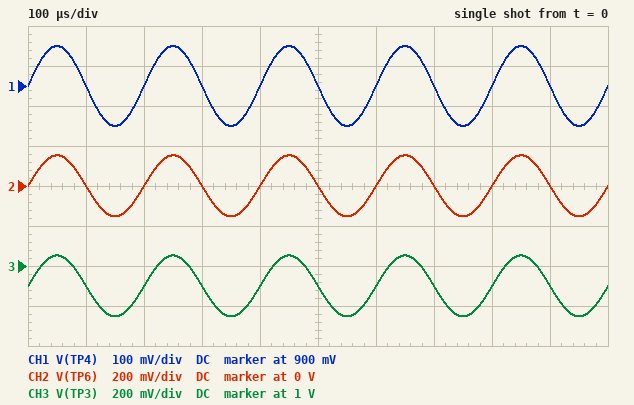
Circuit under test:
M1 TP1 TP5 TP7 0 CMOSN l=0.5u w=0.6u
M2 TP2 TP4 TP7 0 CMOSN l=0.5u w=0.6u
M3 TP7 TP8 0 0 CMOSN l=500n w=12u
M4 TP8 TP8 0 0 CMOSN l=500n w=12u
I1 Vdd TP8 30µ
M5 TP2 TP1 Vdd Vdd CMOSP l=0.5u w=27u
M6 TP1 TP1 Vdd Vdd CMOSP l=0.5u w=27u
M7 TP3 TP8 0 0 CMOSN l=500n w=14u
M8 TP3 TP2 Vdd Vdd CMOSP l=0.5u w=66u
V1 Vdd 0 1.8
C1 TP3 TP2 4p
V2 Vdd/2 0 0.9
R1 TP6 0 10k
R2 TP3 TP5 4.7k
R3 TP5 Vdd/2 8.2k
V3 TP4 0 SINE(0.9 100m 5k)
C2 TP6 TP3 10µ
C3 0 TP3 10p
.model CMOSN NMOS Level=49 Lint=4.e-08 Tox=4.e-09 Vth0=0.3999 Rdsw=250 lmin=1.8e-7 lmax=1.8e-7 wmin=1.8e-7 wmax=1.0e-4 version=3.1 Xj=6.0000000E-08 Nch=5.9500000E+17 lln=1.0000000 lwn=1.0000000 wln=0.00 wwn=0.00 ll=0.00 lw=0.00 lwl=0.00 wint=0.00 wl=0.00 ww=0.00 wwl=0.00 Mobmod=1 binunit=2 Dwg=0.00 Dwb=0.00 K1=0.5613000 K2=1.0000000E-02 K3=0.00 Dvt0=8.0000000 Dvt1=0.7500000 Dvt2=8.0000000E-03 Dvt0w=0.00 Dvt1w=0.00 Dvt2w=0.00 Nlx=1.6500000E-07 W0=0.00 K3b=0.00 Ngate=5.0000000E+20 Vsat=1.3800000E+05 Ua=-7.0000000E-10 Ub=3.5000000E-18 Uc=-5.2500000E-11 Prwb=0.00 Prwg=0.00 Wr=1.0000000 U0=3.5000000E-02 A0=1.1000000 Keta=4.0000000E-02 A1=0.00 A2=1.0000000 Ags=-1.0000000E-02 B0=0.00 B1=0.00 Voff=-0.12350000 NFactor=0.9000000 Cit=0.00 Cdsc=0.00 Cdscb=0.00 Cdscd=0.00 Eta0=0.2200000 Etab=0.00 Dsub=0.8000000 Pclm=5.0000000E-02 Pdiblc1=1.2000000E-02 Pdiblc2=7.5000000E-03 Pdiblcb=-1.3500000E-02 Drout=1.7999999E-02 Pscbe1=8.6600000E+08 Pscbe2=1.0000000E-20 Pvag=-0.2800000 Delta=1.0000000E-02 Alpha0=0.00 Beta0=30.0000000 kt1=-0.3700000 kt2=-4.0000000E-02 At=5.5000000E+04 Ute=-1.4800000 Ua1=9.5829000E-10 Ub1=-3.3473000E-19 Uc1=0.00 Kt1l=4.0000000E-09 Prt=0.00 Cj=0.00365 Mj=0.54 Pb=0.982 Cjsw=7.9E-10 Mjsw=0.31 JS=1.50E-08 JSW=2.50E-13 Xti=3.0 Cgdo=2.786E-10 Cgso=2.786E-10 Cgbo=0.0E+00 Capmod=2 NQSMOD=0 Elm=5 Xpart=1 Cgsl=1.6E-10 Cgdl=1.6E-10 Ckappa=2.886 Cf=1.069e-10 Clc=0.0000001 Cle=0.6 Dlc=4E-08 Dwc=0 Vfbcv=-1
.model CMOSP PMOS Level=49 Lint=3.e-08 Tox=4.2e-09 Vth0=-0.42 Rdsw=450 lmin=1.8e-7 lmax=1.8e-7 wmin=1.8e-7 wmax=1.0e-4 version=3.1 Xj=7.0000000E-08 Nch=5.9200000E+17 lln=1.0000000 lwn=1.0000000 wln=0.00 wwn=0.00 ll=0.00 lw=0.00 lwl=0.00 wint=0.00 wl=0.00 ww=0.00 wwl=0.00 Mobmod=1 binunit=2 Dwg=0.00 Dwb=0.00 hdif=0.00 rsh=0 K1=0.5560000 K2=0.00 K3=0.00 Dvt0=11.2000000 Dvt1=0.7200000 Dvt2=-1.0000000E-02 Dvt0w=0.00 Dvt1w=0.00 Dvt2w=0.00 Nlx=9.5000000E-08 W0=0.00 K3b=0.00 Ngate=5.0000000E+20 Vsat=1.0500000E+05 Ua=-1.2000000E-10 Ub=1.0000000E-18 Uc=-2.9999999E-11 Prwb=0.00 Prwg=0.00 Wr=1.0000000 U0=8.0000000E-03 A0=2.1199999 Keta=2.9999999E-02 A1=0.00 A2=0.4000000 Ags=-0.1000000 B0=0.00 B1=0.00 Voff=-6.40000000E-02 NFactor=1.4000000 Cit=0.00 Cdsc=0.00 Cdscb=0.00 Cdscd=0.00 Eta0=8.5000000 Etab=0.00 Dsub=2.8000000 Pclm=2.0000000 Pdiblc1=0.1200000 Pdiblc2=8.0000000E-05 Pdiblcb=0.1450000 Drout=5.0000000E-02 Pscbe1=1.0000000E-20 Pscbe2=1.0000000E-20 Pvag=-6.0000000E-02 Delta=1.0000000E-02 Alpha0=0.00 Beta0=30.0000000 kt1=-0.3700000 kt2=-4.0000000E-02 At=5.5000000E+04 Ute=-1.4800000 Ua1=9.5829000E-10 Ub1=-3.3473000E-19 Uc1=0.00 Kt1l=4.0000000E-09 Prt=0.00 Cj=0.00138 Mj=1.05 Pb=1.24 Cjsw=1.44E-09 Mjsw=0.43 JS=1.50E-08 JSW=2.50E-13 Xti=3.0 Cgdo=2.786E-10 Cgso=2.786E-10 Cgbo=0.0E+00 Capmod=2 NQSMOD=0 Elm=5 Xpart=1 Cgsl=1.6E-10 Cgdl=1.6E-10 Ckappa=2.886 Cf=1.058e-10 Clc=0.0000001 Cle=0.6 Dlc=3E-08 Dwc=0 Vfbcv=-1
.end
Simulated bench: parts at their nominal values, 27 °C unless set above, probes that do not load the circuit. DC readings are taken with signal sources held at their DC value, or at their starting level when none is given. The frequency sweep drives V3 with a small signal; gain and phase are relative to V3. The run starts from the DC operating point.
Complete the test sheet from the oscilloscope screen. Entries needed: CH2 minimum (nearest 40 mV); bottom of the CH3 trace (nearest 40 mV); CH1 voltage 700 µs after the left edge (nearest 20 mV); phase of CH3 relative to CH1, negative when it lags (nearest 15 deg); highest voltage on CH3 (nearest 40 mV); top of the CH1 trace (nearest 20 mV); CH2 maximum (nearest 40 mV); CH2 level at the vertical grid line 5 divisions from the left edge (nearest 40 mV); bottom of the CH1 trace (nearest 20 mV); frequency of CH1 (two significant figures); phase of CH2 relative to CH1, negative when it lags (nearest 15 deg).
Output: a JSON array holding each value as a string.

["-160 mV", "760 mV", "900 mV", "0 deg", "1.04 V", "1.00 V", "160 mV", "0 V", "800 mV", "5.0 kHz", "0 deg"]
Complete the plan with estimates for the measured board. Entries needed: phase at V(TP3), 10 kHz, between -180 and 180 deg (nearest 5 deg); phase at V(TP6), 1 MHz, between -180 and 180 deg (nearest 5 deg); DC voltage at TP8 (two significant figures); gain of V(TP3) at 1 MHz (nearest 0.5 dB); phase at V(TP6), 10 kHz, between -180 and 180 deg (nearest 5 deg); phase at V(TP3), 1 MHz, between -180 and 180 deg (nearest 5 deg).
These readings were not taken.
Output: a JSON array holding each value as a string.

["0 deg", "-35 deg", "550 mV", "2.5 dB", "0 deg", "-35 deg"]
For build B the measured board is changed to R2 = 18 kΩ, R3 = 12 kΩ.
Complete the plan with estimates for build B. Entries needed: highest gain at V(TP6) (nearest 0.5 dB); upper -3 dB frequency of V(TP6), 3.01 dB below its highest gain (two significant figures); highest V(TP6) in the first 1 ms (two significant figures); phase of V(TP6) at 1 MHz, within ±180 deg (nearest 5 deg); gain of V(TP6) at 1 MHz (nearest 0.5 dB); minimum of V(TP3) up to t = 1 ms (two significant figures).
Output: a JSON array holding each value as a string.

["7.5 dB", "1.1 MHz", "240 mV", "-50 deg", "5.0 dB", "660 mV"]
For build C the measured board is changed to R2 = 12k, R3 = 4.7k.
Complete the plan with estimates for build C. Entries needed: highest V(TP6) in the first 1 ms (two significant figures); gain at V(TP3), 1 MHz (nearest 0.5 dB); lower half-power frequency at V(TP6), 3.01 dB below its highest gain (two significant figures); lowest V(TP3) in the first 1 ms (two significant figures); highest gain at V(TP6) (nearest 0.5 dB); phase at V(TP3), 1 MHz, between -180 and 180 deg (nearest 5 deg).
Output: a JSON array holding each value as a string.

["340 mV", "6.0 dB", "1.5 Hz", "670 mV", "10.5 dB", "-60 deg"]
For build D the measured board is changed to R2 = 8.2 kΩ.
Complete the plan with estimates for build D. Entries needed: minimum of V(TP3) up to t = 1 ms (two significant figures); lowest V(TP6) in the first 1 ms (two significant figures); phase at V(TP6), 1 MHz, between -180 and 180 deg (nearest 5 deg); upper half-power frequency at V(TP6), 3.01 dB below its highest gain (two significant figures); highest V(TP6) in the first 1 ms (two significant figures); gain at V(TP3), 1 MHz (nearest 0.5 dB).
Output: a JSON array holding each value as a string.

["710 mV", "-190 mV", "-45 deg", "1.4 MHz", "190 mV", "4.0 dB"]
